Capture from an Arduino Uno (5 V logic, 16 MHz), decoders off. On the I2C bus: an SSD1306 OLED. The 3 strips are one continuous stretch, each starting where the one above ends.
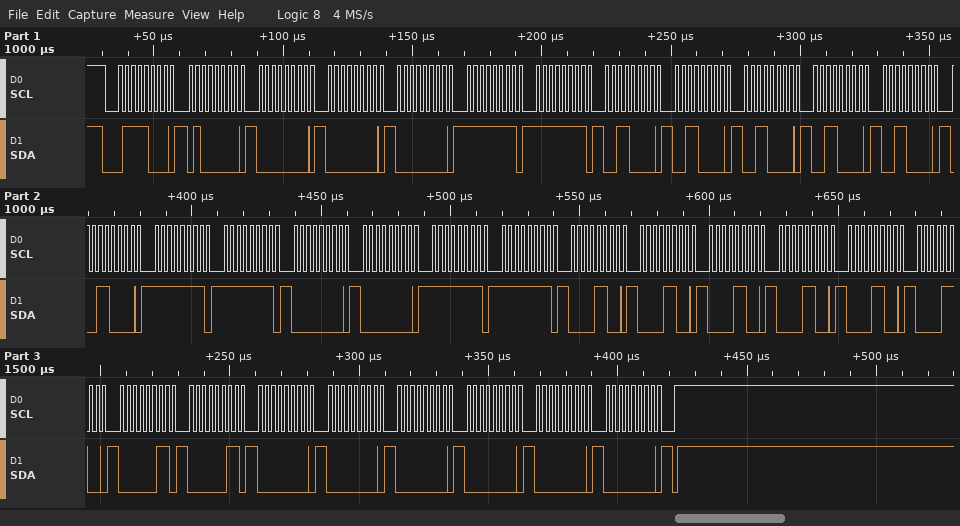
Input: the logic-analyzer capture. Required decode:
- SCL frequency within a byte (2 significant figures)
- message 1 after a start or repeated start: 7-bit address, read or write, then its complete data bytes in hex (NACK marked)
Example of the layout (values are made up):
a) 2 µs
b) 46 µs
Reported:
a) 400 kHz
b) 0x3C write: 40 00 00 00 FF FF 30 30 30 30 30 30 FF FF 00 00 FF FF 0C 0C 0C 0C 0C 0C 03 03 00 00 00 00 00 00
